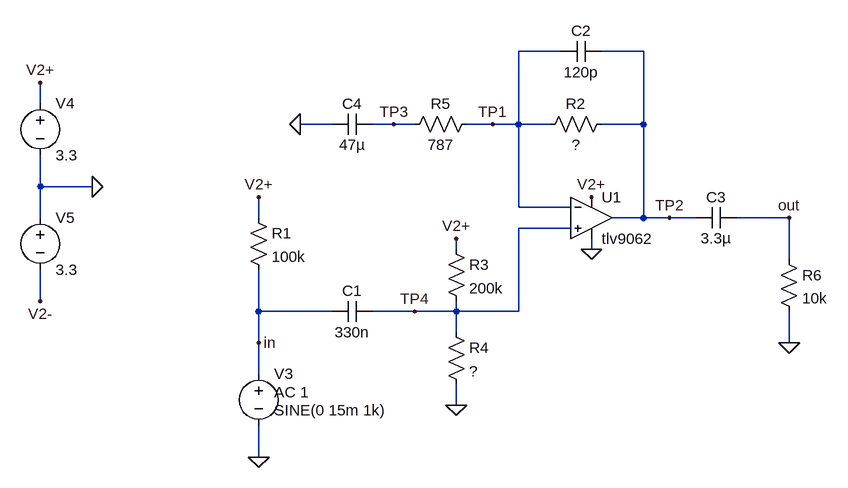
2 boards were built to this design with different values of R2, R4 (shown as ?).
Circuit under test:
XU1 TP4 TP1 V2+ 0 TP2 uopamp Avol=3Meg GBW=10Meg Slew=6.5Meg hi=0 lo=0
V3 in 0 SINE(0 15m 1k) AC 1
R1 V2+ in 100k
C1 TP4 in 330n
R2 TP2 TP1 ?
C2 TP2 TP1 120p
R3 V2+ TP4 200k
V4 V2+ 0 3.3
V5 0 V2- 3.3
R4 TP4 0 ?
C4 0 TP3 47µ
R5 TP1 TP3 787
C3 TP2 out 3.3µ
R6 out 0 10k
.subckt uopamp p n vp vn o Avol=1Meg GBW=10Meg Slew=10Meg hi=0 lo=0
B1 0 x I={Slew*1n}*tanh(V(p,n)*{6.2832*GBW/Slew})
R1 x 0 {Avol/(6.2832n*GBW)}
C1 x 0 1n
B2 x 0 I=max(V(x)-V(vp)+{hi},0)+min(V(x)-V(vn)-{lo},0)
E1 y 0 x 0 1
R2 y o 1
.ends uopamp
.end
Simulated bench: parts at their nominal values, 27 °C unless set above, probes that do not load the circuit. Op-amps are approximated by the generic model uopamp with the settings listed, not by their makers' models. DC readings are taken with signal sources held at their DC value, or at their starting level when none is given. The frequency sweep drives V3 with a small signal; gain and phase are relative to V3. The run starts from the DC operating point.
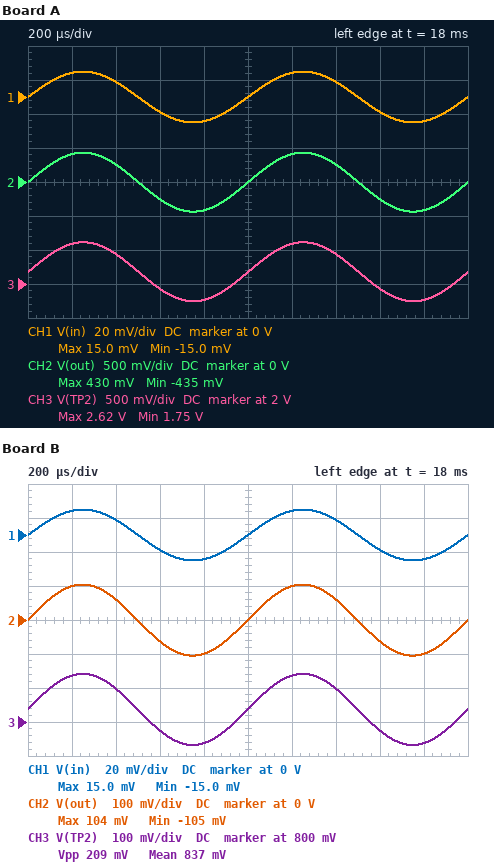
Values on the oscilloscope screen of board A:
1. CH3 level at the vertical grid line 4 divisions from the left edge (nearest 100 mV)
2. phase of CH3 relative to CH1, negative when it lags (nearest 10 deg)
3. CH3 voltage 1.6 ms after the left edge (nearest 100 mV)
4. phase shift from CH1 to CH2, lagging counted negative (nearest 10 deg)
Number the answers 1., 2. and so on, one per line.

1. 1.8 V
2. 0 deg
3. 1.9 V
4. 0 deg
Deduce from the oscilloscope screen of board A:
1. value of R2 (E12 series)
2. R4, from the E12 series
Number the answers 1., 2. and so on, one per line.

1. 22 kΩ
2. 390 kΩ
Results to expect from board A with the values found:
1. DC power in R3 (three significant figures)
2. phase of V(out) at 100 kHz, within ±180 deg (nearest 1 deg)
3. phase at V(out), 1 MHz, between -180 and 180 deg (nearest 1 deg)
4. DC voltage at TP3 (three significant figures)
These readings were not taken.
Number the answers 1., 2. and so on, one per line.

1. 6.26 µW
2. -60 deg
3. -62 deg
4. 2.18 V
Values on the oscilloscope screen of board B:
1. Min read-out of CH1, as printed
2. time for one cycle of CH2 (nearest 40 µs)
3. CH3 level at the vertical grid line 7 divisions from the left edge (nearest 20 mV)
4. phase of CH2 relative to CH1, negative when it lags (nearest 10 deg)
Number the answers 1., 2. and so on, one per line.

1. -15.0 mV
2. 1.00 ms
3. 900 mV
4. 0 deg
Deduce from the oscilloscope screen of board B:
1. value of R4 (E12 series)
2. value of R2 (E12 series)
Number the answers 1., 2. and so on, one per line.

1. 68 kΩ
2. 4.7 kΩ
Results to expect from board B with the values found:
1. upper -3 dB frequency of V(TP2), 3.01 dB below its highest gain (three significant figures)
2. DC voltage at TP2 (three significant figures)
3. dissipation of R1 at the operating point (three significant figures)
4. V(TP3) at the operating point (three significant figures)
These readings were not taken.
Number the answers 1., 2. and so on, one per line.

1. 244 kHz
2. 837 mV
3. 109 µW
4. 837 mV
